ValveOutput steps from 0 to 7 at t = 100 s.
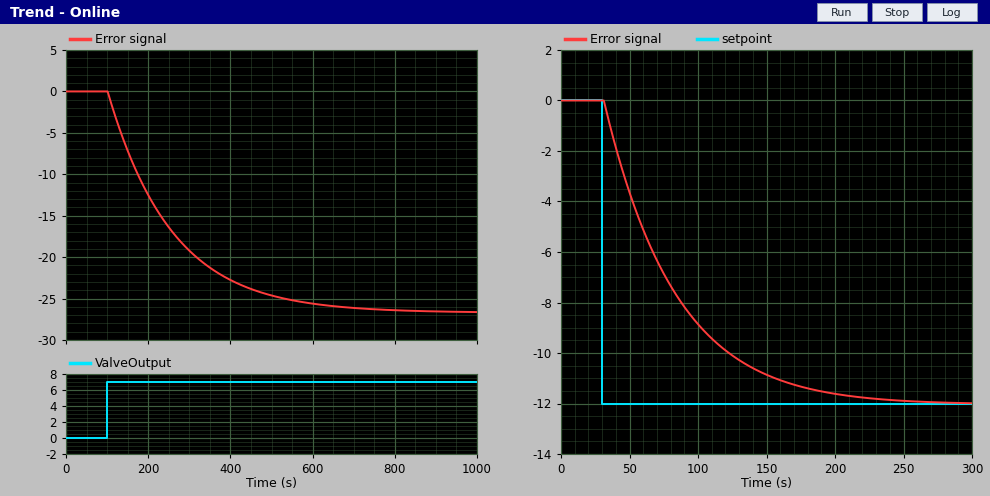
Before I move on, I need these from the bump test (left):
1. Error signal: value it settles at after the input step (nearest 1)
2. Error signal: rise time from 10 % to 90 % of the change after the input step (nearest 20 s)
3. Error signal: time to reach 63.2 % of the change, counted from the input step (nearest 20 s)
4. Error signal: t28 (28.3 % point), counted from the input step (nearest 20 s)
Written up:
-27
340 s
160 s
60 s
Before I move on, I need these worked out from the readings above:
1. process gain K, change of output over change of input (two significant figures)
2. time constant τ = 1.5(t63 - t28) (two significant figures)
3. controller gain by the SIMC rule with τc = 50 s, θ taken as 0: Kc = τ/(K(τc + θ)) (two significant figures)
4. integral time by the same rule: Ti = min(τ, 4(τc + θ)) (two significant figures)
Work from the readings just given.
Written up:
-3.9
150 s
-0.77
150 s
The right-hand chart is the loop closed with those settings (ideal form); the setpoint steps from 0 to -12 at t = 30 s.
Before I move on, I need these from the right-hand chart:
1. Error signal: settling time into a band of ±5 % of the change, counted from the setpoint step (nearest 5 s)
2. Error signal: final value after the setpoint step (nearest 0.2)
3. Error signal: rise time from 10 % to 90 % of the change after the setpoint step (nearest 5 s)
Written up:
150 s
-12.0
110 s
